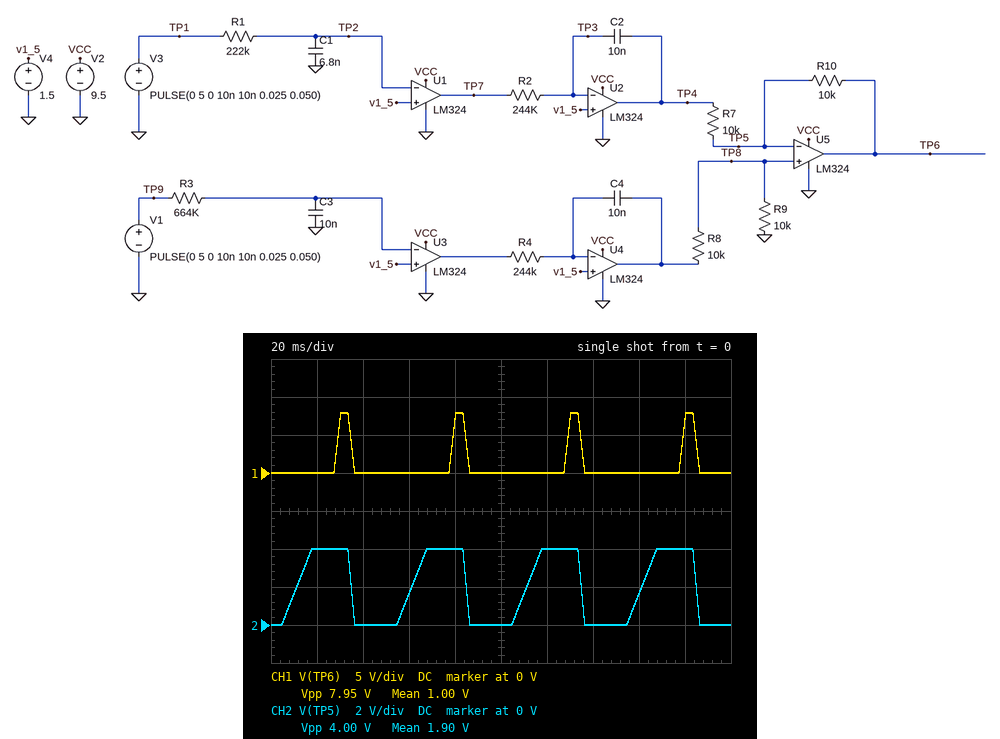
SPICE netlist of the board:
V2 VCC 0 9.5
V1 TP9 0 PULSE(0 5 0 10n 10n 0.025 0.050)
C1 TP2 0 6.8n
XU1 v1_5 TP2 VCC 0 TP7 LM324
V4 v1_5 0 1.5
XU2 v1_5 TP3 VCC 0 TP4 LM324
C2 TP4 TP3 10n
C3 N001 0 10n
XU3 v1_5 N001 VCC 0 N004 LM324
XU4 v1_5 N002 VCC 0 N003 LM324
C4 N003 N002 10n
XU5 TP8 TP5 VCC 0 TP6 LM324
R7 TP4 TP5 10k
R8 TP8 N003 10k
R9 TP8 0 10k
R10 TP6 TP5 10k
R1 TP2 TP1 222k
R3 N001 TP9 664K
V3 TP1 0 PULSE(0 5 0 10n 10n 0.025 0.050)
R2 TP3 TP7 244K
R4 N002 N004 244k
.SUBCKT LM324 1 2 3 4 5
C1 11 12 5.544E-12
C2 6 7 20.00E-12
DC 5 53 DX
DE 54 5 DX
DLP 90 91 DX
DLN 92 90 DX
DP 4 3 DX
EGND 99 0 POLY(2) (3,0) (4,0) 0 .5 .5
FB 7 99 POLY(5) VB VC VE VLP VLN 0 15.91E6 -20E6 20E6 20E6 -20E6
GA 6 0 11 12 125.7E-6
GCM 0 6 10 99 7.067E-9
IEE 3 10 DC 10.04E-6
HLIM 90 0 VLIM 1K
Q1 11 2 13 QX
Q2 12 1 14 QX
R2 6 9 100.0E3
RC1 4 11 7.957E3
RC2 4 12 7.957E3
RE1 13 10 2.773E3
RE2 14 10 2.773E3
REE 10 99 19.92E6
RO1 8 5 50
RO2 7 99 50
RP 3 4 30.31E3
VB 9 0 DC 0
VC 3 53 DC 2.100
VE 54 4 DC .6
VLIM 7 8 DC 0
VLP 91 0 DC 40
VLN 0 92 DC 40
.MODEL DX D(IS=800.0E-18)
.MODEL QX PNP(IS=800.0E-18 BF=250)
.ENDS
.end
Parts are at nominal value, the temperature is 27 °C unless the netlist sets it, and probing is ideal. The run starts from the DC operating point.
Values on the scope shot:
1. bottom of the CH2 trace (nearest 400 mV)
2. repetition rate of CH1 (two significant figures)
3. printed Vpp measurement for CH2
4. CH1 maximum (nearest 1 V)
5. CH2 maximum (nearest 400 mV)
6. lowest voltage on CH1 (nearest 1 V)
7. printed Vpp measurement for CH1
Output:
0 V
20 Hz
4.00 V
8 V
4.0 V
0 V
7.95 V
